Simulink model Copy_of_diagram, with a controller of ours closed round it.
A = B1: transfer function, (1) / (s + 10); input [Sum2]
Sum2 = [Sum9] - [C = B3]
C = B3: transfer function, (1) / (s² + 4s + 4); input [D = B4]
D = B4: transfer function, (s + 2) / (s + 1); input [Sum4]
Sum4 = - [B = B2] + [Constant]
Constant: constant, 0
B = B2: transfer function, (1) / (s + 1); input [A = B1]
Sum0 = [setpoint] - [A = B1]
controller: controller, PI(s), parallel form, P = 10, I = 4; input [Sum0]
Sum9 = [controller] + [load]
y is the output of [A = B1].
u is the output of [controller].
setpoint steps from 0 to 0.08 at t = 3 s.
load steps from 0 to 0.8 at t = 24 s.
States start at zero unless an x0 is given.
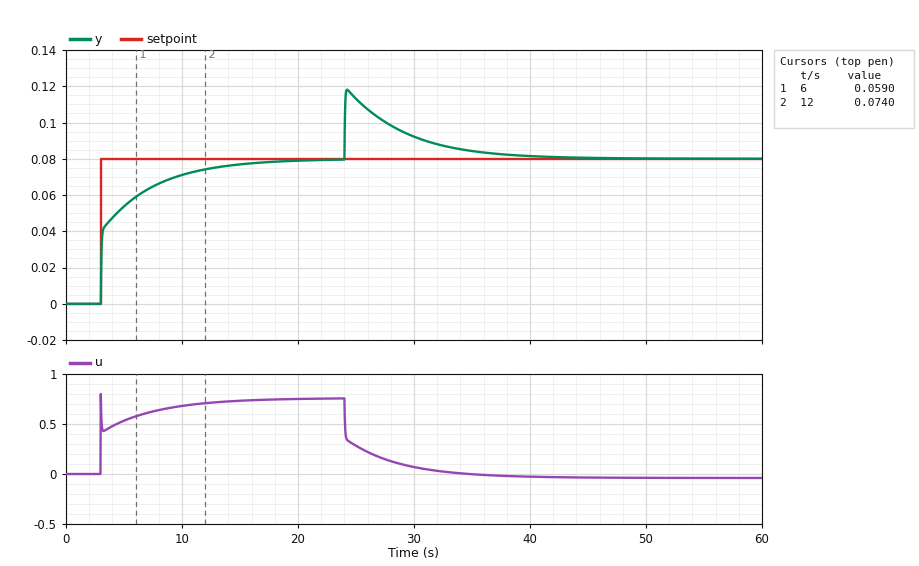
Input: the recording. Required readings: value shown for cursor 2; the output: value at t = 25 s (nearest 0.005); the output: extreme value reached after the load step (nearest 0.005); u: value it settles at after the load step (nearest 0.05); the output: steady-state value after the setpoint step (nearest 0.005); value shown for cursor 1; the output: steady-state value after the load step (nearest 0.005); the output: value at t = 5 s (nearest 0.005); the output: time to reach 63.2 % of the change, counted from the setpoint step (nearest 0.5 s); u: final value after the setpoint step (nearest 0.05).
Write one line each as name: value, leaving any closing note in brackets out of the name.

value shown for cursor 2: 0.0740
the output: value at t = 25 s: 0.115
the output: extreme value reached after the load step: 0.120
u: value it settles at after the load step: -0.05
the output: steady-state value after the setpoint step: 0.080
value shown for cursor 1: 0.0590
the output: steady-state value after the load step: 0.080
the output: value at t = 5 s: 0.055
the output: time to reach 63.2 % of the change, counted from the setpoint step: 1.5 s
u: final value after the setpoint step: 0.75
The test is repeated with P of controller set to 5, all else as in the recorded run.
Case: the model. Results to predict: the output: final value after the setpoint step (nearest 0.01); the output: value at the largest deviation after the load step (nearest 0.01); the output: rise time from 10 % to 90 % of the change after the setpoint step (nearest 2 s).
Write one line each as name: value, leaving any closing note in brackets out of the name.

the output: final value after the setpoint step: 0.08
the output: value at the largest deviation after the load step: 0.13
the output: rise time from 10 % to 90 % of the change after the setpoint step: 6 s
